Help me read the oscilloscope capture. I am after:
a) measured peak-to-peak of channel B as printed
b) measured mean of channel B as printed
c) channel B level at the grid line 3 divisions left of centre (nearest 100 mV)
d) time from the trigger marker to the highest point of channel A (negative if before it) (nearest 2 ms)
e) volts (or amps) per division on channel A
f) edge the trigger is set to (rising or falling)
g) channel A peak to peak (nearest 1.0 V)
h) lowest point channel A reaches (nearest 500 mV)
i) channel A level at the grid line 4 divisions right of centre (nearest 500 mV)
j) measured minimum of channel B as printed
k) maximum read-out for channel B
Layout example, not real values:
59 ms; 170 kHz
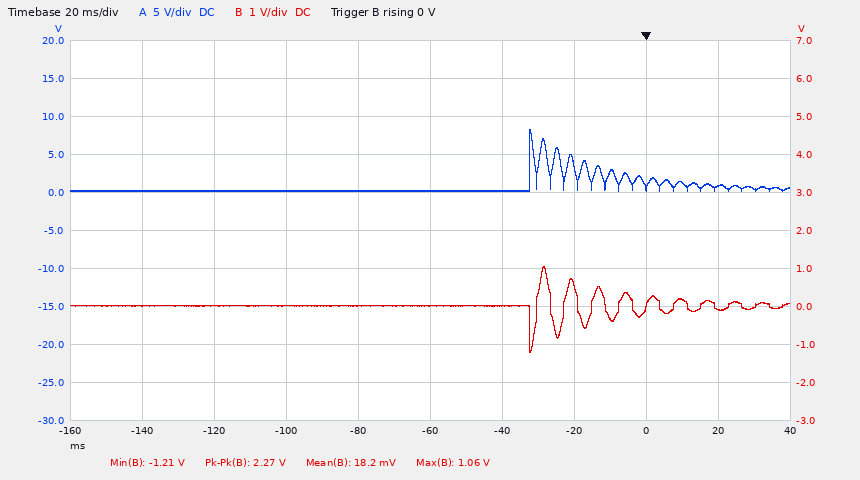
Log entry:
2.27 V; 18.2 mV; 0.0 V; -32 ms; 5 V; rising; 8.0 V; 0.0 V; 1.0 V; -1.21 V; 1.06 V
